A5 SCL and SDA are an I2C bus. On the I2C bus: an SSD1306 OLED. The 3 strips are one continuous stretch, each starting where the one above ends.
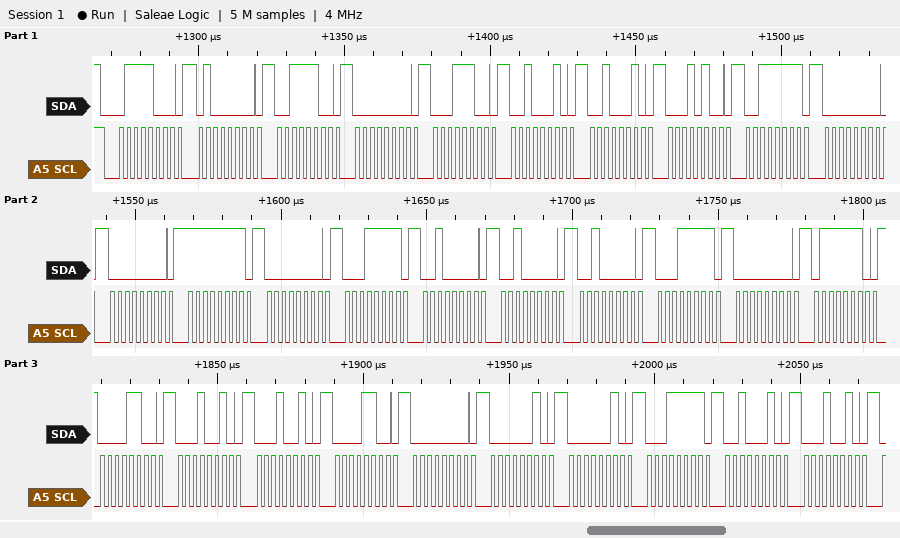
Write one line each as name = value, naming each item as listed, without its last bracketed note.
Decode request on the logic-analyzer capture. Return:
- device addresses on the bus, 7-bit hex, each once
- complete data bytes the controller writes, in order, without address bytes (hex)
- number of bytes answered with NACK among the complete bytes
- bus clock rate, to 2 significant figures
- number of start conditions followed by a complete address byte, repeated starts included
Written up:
device addresses on the bus, 7-bit hex, each once = 0x3C
complete data bytes the controller writes, in order, without address bytes = 40 3C 00 1C 22 22 14 3F 00 00 FF 00 1F 20 20 20 1F 00 7E 0C 12 12 0C 00 02 02 1F 22 12
number of bytes answered with NACK among the complete bytes = 0
bus clock rate, to 2 significant figures = 400 kHz
number of start conditions followed by a complete address byte, repeated starts included = 1
